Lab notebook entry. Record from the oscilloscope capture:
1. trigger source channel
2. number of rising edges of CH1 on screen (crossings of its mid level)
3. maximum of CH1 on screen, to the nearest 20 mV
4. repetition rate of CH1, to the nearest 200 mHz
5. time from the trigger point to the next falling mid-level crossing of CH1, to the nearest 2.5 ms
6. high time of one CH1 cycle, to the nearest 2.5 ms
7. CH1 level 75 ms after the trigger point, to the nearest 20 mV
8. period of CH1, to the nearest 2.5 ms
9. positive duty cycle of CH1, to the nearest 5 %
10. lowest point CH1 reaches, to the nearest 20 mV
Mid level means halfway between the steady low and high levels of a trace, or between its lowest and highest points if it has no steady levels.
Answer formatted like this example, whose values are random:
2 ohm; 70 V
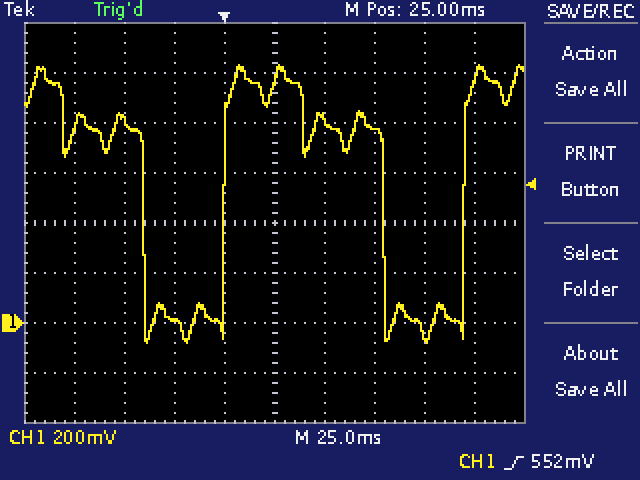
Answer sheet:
CH1; 2; 1.04 V; 8.4 Hz; 80.0 ms; 80.0 ms; 780 mV; 120.0 ms; 65 %; -80 mV
